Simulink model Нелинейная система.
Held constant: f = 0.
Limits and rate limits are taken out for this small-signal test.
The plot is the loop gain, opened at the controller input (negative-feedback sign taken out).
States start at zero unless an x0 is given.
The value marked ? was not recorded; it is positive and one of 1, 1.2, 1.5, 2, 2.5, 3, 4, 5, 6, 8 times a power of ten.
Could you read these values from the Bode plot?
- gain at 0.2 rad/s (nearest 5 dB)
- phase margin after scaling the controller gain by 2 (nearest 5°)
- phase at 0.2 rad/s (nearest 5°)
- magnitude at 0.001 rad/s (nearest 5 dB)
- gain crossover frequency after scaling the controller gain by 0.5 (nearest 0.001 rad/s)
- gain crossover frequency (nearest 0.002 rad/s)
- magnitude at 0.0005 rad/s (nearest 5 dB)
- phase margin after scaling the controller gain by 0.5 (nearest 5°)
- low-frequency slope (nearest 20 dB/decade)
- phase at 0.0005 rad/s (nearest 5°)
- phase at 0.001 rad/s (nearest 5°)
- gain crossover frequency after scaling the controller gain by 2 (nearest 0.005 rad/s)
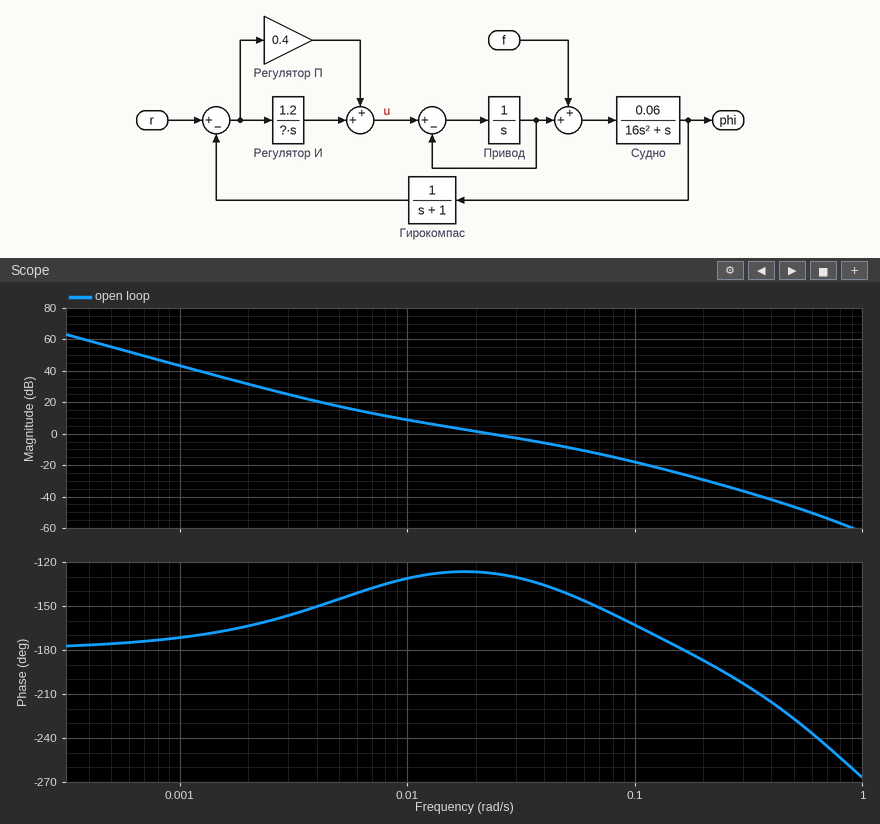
-30 dB
45°
-185°
45 dB
0.013 rad/s
0.024 rad/s
55 dB
50°
-40 dB/decade
-175°
-170°
0.040 rad/s
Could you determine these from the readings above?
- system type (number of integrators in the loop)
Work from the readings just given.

2
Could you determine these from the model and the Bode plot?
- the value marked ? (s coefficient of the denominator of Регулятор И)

500
